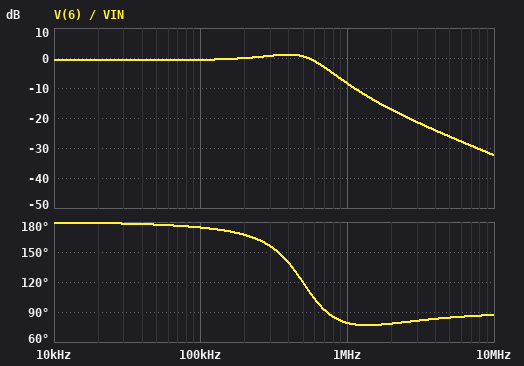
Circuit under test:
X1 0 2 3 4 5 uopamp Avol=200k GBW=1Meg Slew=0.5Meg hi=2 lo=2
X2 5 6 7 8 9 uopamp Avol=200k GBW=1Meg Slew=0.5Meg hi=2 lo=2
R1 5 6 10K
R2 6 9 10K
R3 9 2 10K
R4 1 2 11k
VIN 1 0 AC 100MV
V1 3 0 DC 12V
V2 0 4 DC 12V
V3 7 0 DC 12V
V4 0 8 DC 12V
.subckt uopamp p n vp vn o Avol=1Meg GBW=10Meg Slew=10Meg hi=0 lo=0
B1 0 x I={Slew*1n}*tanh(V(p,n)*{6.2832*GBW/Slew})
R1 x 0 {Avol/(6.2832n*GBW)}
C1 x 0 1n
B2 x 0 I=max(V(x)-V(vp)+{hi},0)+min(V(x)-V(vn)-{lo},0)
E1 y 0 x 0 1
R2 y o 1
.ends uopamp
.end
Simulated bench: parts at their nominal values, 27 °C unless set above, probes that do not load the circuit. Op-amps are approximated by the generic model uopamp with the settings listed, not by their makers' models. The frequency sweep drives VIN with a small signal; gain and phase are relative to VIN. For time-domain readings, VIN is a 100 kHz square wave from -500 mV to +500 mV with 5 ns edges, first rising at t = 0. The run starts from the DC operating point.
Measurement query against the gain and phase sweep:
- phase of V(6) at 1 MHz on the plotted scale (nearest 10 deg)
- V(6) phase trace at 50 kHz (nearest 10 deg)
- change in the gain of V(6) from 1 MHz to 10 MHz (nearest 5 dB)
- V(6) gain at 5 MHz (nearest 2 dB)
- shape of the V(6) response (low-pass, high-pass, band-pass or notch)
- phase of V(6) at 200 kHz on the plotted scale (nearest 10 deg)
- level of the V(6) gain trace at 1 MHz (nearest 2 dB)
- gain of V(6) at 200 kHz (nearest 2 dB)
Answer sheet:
80 deg
180 deg
-25 dB
-26 dB
low-pass
170 deg
-8 dB
0 dB
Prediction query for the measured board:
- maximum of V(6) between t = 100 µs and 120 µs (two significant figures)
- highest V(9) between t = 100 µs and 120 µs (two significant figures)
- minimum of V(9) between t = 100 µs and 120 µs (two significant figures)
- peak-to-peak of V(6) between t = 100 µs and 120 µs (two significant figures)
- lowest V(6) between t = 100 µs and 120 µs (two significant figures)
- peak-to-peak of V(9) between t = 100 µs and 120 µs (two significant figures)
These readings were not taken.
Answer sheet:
550 mV
540 mV
-540 mV
1.1 V
-550 mV
1.1 V
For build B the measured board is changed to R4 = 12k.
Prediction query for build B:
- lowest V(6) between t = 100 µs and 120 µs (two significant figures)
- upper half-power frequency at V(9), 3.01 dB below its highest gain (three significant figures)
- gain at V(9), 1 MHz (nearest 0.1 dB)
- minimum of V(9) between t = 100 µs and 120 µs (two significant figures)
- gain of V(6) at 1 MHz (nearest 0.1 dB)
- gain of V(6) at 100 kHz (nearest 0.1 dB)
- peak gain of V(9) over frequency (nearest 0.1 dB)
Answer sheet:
-510 mV
614 kHz
-11.8 dB
-500 mV
-8.8 dB
-1.4 dB
-0.1 dB
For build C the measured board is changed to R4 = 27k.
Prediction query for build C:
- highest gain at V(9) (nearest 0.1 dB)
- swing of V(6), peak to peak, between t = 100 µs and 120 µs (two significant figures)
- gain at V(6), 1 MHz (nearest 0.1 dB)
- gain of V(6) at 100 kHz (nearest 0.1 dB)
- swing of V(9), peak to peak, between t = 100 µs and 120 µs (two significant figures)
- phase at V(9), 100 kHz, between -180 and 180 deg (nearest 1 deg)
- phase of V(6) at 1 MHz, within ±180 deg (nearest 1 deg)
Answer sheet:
-6.2 dB
520 mV
-12.5 dB
-8.4 dB
490 mV
172 deg
83 deg
